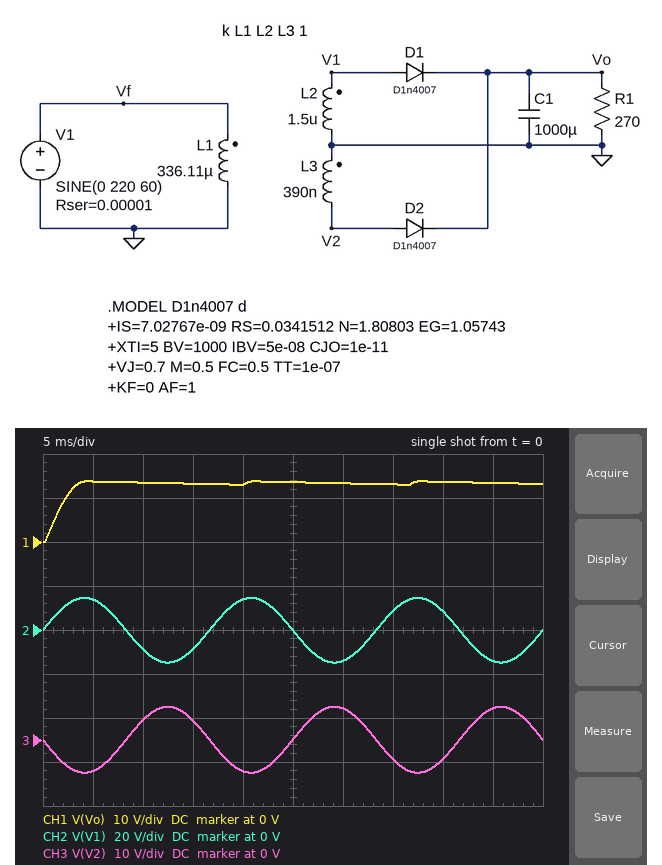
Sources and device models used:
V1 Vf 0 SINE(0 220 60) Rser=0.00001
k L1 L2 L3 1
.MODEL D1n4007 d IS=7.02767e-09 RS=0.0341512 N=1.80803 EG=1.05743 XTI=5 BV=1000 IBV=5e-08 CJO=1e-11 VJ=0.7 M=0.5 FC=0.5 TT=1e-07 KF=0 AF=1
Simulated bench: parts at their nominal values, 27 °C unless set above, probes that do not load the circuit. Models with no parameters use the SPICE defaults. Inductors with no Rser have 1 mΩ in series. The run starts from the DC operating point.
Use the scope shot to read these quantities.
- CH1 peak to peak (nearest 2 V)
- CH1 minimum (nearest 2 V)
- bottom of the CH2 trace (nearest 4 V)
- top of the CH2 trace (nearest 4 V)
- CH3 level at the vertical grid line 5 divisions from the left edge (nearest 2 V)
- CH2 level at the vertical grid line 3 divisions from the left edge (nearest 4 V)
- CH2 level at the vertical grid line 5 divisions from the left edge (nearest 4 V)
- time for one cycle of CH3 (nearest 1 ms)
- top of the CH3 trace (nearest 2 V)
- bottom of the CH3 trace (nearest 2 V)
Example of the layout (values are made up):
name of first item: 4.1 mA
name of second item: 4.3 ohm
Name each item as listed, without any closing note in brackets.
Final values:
CH1 peak to peak: 14 V
CH1 minimum: 0 V
bottom of the CH2 trace: -16 V
top of the CH2 trace: 16 V
CH3 level at the vertical grid line 5 divisions from the left edge: 0 V
CH2 level at the vertical grid line 3 divisions from the left edge: -8 V
CH2 level at the vertical grid line 5 divisions from the left edge: 0 V
time for one cycle of CH3: 17 ms
top of the CH3 trace: 8 V
bottom of the CH3 trace: -8 V
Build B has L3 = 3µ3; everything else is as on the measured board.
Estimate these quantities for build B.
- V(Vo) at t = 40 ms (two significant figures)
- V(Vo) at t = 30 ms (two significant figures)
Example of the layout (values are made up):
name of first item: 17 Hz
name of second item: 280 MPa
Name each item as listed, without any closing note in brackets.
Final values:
V(Vo) at t = 40 ms: 20 V
V(Vo) at t = 30 ms: 21 V
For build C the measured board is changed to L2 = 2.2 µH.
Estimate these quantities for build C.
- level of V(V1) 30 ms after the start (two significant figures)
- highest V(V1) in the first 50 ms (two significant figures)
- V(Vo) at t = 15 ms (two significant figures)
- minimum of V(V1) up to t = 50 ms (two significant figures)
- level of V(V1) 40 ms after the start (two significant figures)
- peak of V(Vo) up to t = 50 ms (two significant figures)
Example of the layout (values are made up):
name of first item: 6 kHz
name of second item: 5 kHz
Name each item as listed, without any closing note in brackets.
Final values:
level of V(V1) 30 ms after the start: -17 V
highest V(V1) in the first 50 ms: 18 V
V(Vo) at t = 15 ms: 16 V
minimum of V(V1) up to t = 50 ms: -18 V
level of V(V1) 40 ms after the start: 10 V
peak of V(Vo) up to t = 50 ms: 17 V
